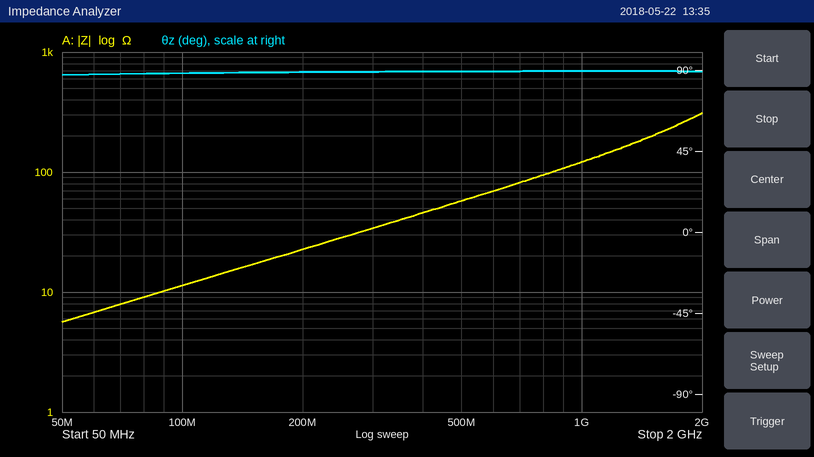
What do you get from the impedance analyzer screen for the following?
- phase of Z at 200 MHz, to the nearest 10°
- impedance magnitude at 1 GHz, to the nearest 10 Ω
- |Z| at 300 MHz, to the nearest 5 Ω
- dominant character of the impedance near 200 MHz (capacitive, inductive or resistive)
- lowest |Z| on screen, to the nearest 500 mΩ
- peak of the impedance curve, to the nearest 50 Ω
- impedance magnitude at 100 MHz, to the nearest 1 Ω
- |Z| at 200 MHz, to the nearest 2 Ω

90°
120 Ω
35 Ω
inductive
5.5 Ω
300 Ω
11 Ω
22 Ω
